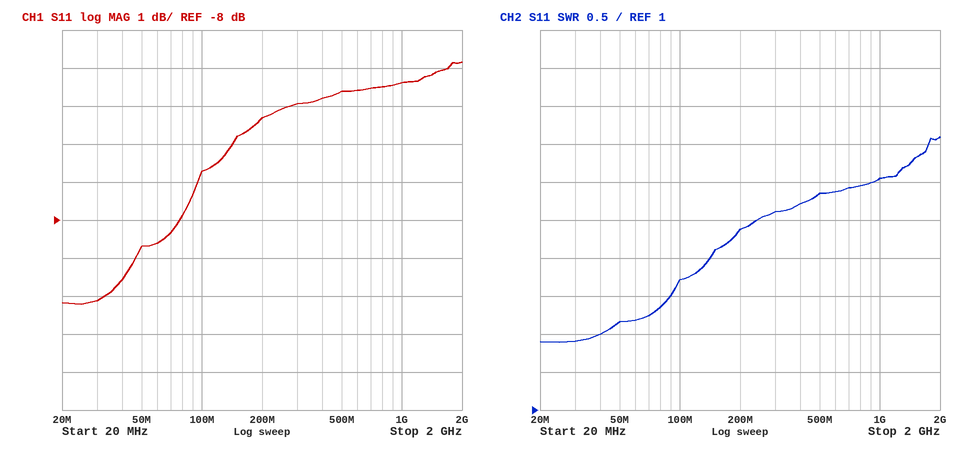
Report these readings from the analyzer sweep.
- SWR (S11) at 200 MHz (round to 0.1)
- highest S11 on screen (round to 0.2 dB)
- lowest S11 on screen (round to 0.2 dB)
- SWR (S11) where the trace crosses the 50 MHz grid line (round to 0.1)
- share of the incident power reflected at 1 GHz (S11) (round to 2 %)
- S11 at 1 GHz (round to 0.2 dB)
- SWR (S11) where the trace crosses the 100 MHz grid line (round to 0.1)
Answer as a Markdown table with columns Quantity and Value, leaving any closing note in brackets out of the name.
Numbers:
| Quantity | Value |
|---|---|
| SWR (S11) at 200 MHz | 3.4 |
| highest S11 on screen | -3.8 dB |
| lowest S11 on screen | -10.2 dB |
| SWR (S11) where the trace crosses the 50 MHz grid line | 2.2 |
| share of the incident power reflected at 1 GHz (S11) | 36 % |
| S11 at 1 GHz | -4.4 dB |
| SWR (S11) where the trace crosses the 100 MHz grid line | 2.7 |
